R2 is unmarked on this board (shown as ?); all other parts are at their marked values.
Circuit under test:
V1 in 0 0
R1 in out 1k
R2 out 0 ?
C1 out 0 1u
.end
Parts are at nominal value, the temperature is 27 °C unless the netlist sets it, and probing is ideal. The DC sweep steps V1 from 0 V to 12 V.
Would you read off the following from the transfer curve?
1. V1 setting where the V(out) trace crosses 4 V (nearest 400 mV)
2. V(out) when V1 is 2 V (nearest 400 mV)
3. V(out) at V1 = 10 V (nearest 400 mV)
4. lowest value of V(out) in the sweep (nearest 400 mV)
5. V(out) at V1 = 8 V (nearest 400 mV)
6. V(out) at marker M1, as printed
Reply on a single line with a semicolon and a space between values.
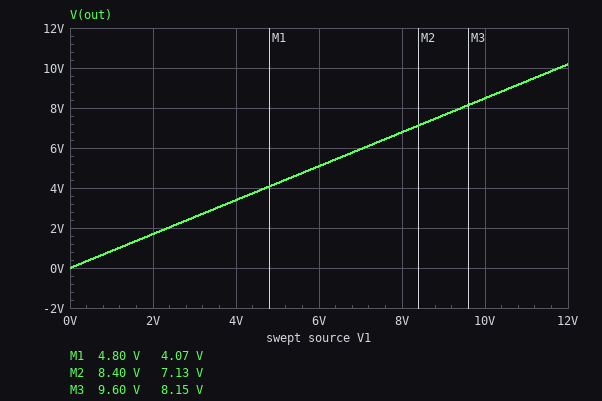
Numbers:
4.8 V; 1.6 V; 8.4 V; 0 V; 6.8 V; 4.07 V
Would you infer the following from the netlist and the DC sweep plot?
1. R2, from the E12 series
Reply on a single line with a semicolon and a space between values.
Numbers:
5.6 kΩ
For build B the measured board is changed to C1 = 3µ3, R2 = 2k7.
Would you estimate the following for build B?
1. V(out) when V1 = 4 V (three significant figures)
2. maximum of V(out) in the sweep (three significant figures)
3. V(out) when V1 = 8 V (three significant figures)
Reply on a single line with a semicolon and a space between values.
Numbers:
2.92 V; 8.76 V; 5.84 V
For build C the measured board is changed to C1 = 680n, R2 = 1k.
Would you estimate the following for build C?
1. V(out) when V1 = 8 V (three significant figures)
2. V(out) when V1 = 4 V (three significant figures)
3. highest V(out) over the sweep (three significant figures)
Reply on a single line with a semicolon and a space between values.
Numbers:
4.00 V; 2.00 V; 6.00 V
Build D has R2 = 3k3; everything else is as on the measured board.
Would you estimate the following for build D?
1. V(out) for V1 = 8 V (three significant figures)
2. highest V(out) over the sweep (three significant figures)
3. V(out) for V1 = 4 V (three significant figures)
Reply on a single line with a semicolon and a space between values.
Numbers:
6.14 V; 9.21 V; 3.07 V
